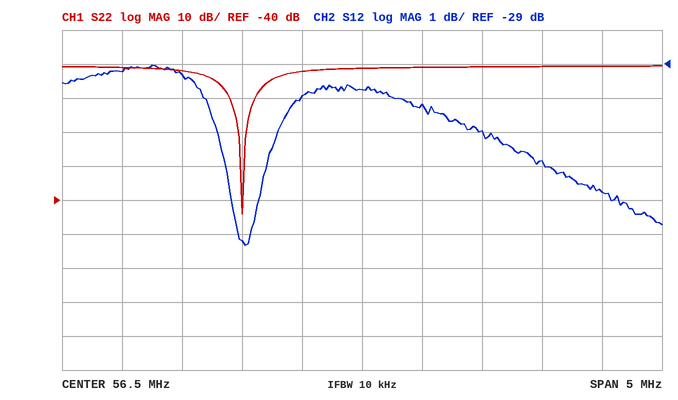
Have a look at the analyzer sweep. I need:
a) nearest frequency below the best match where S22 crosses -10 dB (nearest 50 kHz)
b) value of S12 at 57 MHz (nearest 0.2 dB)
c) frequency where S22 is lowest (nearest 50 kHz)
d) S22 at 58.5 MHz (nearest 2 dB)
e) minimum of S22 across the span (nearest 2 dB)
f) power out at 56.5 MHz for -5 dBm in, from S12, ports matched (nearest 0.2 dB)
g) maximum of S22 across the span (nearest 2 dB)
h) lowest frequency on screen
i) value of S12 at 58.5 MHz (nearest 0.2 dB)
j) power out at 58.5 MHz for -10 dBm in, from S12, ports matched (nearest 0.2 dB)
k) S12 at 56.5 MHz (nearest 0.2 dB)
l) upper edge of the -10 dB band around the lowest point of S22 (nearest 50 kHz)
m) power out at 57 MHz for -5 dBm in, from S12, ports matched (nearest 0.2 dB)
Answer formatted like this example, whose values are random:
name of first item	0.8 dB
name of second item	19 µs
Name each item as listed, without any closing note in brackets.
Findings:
nearest frequency below the best match where S22 crosses -10 dB	55.40 MHz
value of S12 at 57 MHz	-30.2 dB
frequency where S22 is lowest	55.50 MHz
S22 at 58.5 MHz	0 dB
minimum of S22 across the span	-44 dB
power out at 56.5 MHz for -5 dBm in, from S12, ports matched	-34.8 dBm
maximum of S22 across the span	0 dB
lowest frequency on screen	54 MHz
value of S12 at 58.5 MHz	-32.8 dB
power out at 58.5 MHz for -10 dBm in, from S12, ports matched	-42.8 dBm
S12 at 56.5 MHz	-29.8 dB
upper edge of the -10 dB band around the lowest point of S22	55.60 MHz
power out at 57 MHz for -5 dBm in, from S12, ports matched	-35.2 dBm
